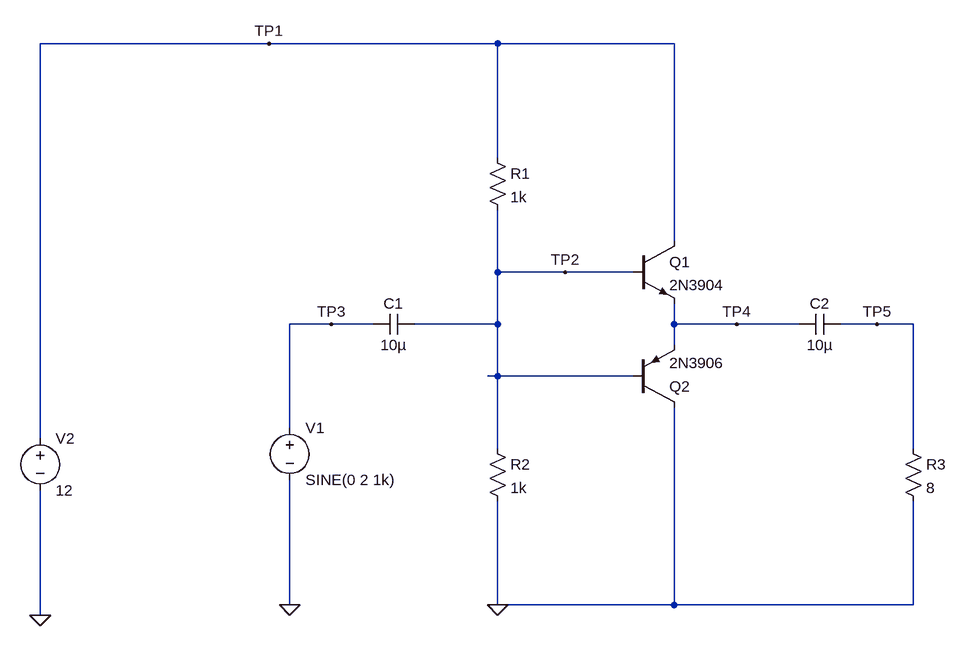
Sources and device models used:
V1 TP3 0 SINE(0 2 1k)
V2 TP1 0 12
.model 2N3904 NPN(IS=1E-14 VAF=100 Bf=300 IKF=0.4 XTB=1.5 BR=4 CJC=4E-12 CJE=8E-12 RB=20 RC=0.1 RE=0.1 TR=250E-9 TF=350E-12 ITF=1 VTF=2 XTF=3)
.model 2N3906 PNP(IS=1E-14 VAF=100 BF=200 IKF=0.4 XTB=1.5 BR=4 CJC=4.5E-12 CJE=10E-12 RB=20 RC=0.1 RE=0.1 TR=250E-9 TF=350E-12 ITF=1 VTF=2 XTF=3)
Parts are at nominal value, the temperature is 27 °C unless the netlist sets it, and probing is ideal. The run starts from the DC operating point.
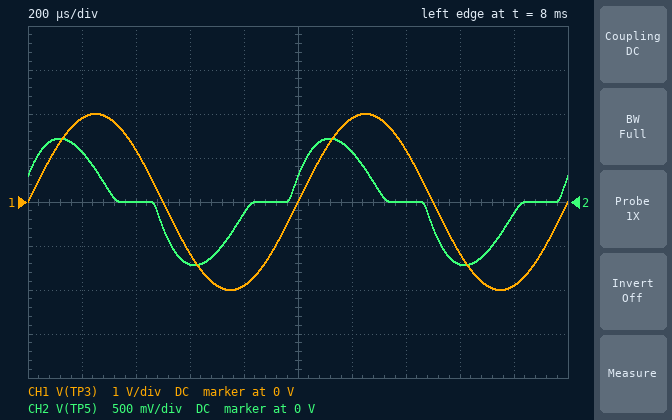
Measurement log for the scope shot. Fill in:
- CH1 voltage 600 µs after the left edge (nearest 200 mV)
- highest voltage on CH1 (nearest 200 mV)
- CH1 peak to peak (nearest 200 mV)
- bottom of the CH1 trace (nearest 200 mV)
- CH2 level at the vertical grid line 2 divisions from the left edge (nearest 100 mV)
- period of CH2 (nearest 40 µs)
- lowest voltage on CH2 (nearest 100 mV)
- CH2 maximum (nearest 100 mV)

-1.2 V
2.0 V
4.0 V
-2.0 V
0 V
1.00 ms
-700 mV
700 mV
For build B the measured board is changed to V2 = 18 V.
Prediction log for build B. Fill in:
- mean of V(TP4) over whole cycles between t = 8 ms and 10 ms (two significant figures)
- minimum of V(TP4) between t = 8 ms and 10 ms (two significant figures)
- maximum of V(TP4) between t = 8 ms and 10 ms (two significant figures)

9.0 V
7.8 V
10 V
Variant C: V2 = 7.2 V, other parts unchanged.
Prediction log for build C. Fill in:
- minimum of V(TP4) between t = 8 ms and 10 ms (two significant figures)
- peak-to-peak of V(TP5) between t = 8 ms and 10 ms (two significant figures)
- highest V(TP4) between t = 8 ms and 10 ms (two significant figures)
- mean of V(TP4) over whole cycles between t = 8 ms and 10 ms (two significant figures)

2.4 V
1.4 V
4.8 V
3.6 V
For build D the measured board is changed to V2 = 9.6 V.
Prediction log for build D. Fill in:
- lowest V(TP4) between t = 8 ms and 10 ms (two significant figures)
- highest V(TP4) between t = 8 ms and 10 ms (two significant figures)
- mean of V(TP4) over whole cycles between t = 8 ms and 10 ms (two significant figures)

3.6 V
6.0 V
4.8 V
